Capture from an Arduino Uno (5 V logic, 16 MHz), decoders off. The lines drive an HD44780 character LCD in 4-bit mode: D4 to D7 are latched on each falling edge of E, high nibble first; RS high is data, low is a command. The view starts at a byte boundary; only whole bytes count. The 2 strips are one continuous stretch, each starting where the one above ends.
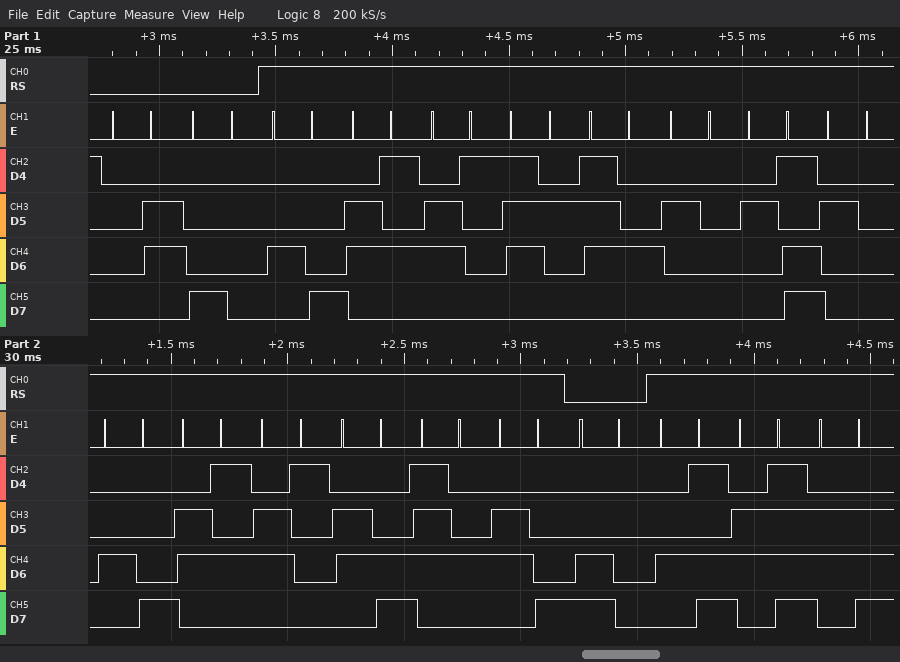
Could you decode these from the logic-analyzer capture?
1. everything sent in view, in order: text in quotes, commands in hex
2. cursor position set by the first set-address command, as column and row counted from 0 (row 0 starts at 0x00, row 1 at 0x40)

0x06 0x80 "Heart - Health" 0xC0 "Mon"
column 0, row 0
